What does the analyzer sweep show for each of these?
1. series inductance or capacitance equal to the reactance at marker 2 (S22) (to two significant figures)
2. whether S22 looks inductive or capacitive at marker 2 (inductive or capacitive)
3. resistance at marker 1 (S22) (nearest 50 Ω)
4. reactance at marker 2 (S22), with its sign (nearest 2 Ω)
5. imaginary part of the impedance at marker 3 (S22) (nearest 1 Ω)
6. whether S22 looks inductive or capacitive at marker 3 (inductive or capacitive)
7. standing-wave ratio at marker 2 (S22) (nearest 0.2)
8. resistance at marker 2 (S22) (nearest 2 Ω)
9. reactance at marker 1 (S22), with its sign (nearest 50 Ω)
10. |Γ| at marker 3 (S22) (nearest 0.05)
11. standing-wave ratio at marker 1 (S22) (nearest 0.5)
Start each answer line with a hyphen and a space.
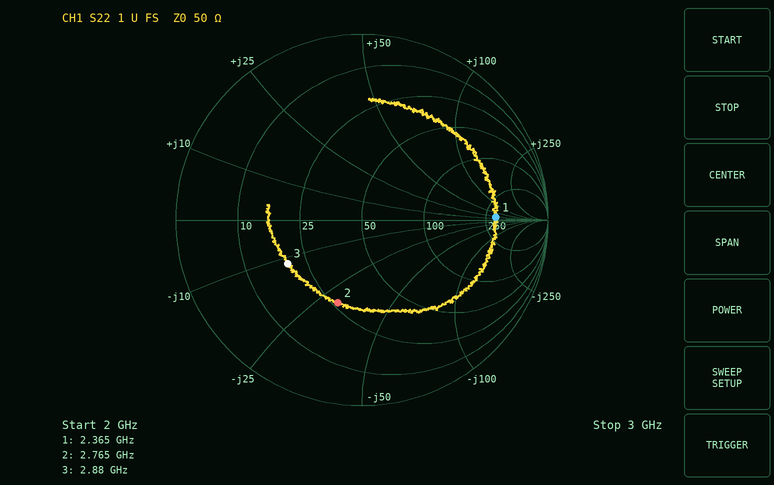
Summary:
- 1.9 pF
- capacitive
- 300 Ω
- -30 Ω
- -12 Ω
- capacitive
- 2.8
- 26 Ω
- 0 Ω
- 0.45
- 6.0
